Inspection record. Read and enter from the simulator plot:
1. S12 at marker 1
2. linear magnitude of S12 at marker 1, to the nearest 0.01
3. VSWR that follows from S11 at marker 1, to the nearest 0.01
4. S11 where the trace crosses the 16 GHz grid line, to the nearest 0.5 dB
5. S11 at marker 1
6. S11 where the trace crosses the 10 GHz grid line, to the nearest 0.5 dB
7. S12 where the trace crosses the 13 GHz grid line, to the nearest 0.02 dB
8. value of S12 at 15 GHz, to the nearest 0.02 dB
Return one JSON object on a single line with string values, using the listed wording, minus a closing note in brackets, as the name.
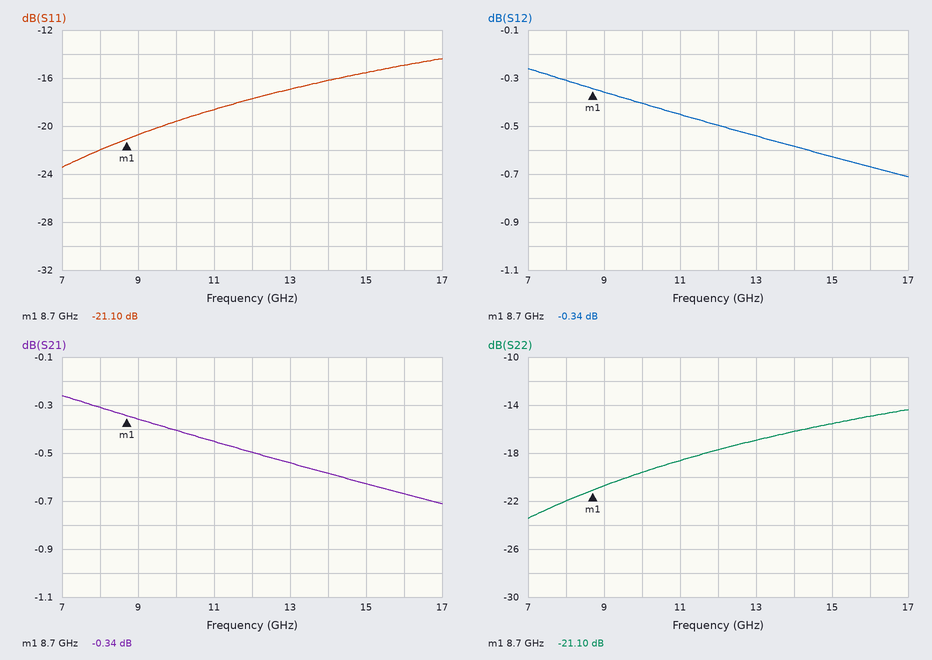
{"S12 at marker 1": "-0.34 dB", "linear magnitude of S12 at marker 1, to the nearest 0.01": "0.96", "VSWR that follows from S11 at marker 1, to the nearest 0.01": "1.19", "S11 where the trace crosses the 16 GHz grid line, to the nearest 0.5 dB": "-15.0 dB", "S11 at marker 1": "-21.10 dB", "S11 where the trace crosses the 10 GHz grid line, to the nearest 0.5 dB": "-19.5 dB", "S12 where the trace crosses the 13 GHz grid line, to the nearest 0.02 dB": "-0.54 dB", "value of S12 at 15 GHz, to the nearest 0.02 dB": "-0.62 dB"}
